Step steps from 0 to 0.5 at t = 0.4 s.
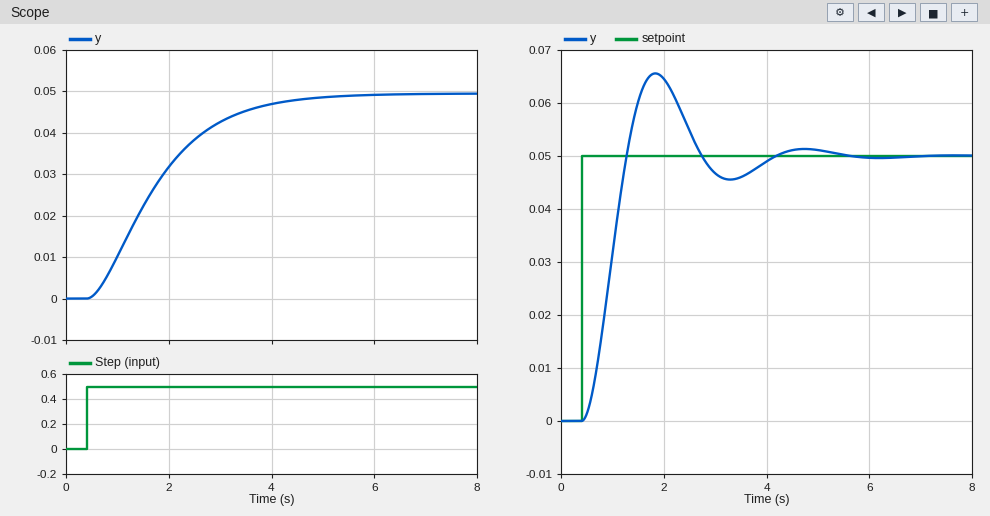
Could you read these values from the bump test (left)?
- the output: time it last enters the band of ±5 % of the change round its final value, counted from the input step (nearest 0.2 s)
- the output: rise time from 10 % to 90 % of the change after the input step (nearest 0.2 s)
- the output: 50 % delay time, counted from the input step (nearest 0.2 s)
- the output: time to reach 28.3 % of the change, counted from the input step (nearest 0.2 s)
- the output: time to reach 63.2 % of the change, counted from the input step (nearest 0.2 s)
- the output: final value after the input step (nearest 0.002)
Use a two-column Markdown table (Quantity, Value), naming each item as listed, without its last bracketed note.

| Quantity | Value |
|---|---|
| the output: time it last enters the band of ±5 % of the change round its final value, counted from the input step | 3.6 s |
| the output: rise time from 10 % to 90 % of the change after the input step | 2.6 s |
| the output: 50 % delay time, counted from the input step | 1.2 s |
| the output: time to reach 28.3 % of the change, counted from the input step | 0.8 s |
| the output: time to reach 63.2 % of the change, counted from the input step | 1.6 s |
| the output: final value after the input step | 0.050 |
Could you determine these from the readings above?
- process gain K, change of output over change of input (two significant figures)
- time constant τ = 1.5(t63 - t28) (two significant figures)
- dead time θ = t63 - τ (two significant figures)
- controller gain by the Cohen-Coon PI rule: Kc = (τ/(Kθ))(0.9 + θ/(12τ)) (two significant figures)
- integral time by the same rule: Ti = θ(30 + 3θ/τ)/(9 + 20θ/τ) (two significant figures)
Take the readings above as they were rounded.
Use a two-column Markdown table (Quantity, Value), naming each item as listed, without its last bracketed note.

| Quantity | Value |
|---|---|
| process gain K, change of output over change of input | 0.10 |
| time constant τ = 1.5(t63 - t28) | 1.2 s |
| dead time θ = t63 - τ | 0.40 s |
| controller gain by the Cohen-Coon PI rule: Kc = (τ/(Kθ))(0.9 + θ/(12τ)) | 28 |
| integral time by the same rule: Ti = θ(30 + 3θ/τ)/(9 + 20θ/τ) | 0.79 s |
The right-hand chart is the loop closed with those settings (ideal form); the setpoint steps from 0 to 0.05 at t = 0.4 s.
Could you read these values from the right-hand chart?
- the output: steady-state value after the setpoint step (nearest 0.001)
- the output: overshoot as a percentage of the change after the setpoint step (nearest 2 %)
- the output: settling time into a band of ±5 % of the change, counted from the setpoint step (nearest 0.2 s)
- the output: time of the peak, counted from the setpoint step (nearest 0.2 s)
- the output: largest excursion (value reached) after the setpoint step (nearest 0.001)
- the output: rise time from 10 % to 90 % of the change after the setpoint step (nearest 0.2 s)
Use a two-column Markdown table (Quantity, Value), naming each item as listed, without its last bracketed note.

| Quantity | Value |
|---|---|
| the output: steady-state value after the setpoint step | 0.050 |
| the output: overshoot as a percentage of the change after the setpoint step | 32 % |
| the output: settling time into a band of ±5 % of the change, counted from the setpoint step | 3.4 s |
| the output: time of the peak, counted from the setpoint step | 1.4 s |
| the output: largest excursion (value reached) after the setpoint step | 0.066 |
| the output: rise time from 10 % to 90 % of the change after the setpoint step | 0.6 s |
